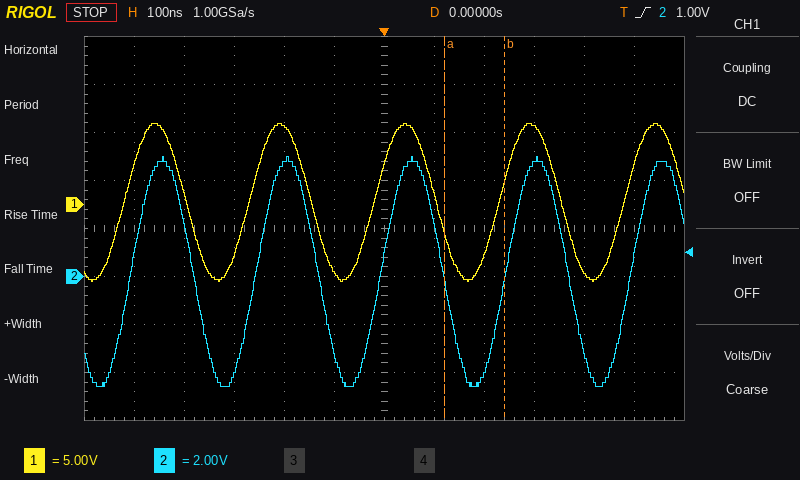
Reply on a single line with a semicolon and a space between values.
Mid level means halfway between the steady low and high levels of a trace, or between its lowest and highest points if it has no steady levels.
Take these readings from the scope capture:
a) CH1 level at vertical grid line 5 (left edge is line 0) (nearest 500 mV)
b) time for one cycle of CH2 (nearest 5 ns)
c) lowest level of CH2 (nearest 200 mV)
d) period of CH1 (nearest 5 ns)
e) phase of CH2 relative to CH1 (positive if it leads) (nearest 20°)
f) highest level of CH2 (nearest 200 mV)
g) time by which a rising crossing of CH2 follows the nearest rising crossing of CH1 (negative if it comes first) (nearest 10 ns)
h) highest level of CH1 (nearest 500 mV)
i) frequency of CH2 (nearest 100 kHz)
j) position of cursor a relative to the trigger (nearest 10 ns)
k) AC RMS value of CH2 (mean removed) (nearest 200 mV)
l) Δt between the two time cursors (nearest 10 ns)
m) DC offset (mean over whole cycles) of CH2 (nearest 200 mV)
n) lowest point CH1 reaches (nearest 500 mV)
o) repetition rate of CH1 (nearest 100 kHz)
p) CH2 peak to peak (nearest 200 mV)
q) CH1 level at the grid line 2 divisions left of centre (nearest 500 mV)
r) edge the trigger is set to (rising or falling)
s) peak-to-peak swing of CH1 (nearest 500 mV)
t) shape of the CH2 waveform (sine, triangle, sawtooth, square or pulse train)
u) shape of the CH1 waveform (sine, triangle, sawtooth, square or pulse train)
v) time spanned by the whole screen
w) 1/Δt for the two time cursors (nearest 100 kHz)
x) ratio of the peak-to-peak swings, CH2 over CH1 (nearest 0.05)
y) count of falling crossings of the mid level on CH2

-7.0 V; 250 ns; -4.6 V; 250 ns; -20°; 5.0 V; +10 ns; 8.5 V; 4.0 MHz; +120 ns; 3.4 V; 120 ns; 200 mV; -8.0 V; 4.0 MHz; 9.6 V; 8.0 V; rising; 16.5 V; sine; sine; 1.2 µs; 8.3 MHz; 0.60; 4
